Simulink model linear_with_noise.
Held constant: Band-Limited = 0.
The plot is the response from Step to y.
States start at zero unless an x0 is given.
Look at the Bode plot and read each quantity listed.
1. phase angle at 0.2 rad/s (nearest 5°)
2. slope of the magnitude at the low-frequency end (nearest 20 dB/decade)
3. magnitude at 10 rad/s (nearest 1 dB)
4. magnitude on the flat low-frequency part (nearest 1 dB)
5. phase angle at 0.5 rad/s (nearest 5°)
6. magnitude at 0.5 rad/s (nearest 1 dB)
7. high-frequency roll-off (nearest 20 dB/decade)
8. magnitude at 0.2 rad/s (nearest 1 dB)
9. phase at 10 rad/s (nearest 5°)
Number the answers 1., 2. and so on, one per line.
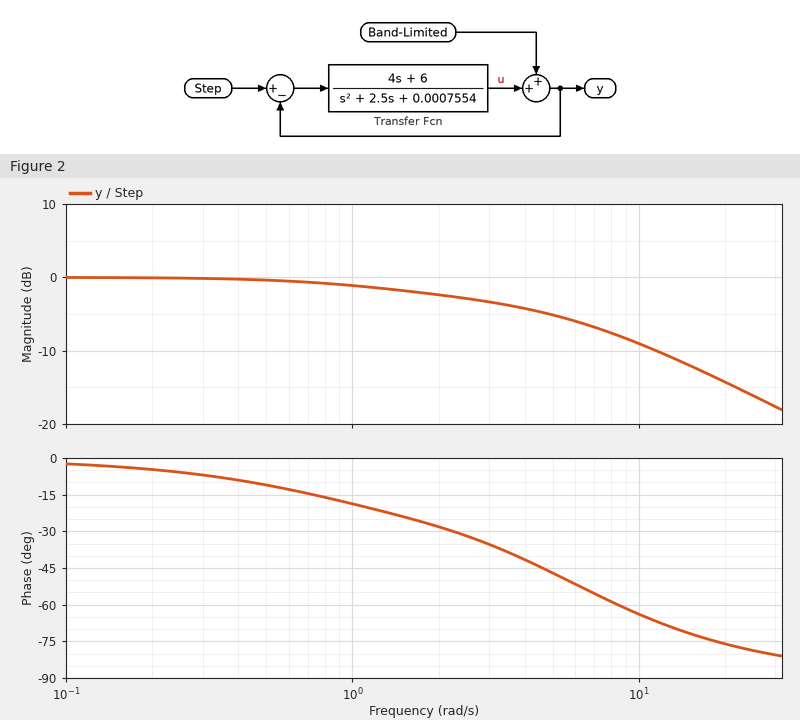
1. -5°
2. 0 dB/decade
3. -9 dB
4. 0 dB
5. -10°
6. 0 dB
7. -20 dB/decade
8. 0 dB
9. -65°
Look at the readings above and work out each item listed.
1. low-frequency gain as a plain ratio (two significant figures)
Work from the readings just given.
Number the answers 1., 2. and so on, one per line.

1. 1.0
